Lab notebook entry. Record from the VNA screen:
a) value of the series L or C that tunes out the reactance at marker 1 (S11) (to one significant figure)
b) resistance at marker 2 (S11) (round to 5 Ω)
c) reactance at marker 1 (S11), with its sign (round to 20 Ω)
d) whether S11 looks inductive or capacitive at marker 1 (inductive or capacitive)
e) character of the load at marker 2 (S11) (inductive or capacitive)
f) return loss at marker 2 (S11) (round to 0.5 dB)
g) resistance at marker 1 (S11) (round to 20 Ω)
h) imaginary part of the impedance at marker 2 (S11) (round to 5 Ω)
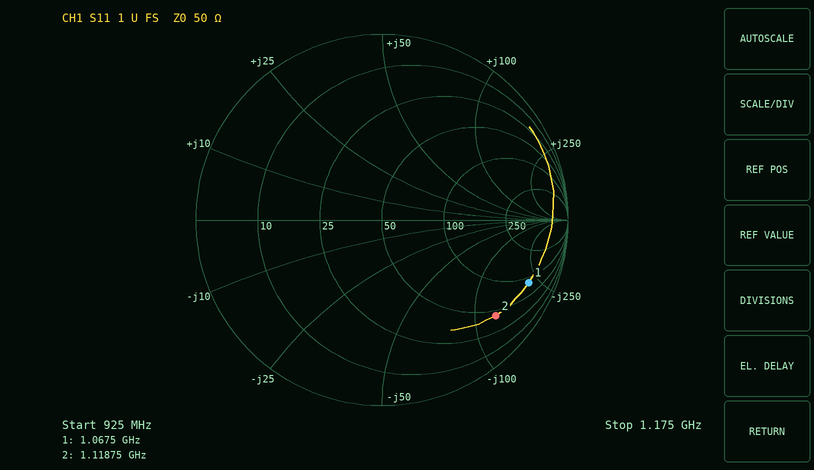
30 nH
45 Ω
-220 Ω
capacitive
capacitive
2.0 dB
80 Ω
-125 Ω
